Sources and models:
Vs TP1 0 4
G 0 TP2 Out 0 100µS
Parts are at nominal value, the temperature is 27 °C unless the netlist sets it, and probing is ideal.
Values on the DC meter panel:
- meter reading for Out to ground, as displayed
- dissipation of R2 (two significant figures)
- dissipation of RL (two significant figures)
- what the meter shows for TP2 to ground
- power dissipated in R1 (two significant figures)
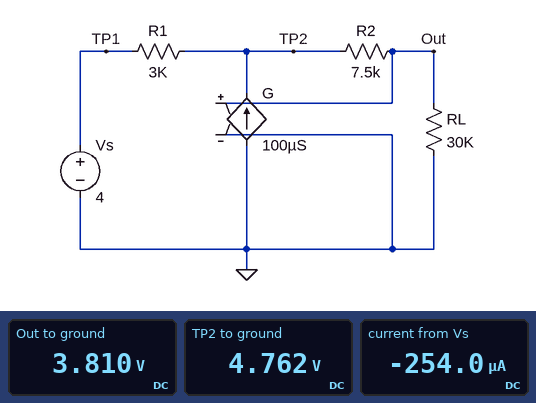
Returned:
3.810 V
120 µW
480 µW
4.762 V
190 µW
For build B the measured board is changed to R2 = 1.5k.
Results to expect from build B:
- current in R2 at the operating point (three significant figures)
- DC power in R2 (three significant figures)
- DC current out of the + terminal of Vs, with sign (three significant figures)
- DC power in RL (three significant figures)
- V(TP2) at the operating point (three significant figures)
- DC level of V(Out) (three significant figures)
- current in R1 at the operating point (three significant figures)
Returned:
157 µA
36.9 µW
-314 µA
738 µW
4.94 V
4.71 V
314 µA
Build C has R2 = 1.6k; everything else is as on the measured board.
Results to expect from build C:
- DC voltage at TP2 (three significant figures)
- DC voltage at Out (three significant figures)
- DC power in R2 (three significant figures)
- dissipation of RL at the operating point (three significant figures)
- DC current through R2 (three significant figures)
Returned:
4.94 V
4.69 V
39.1 µW
732 µW
156 µA
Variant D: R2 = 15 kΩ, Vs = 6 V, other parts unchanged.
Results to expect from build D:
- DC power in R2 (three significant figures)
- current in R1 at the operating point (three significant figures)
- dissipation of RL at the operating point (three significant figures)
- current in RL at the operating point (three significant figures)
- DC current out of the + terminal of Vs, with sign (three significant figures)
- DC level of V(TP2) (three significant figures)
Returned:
355 µW
308 µA
710 µW
154 µA
-308 µA
6.92 V
